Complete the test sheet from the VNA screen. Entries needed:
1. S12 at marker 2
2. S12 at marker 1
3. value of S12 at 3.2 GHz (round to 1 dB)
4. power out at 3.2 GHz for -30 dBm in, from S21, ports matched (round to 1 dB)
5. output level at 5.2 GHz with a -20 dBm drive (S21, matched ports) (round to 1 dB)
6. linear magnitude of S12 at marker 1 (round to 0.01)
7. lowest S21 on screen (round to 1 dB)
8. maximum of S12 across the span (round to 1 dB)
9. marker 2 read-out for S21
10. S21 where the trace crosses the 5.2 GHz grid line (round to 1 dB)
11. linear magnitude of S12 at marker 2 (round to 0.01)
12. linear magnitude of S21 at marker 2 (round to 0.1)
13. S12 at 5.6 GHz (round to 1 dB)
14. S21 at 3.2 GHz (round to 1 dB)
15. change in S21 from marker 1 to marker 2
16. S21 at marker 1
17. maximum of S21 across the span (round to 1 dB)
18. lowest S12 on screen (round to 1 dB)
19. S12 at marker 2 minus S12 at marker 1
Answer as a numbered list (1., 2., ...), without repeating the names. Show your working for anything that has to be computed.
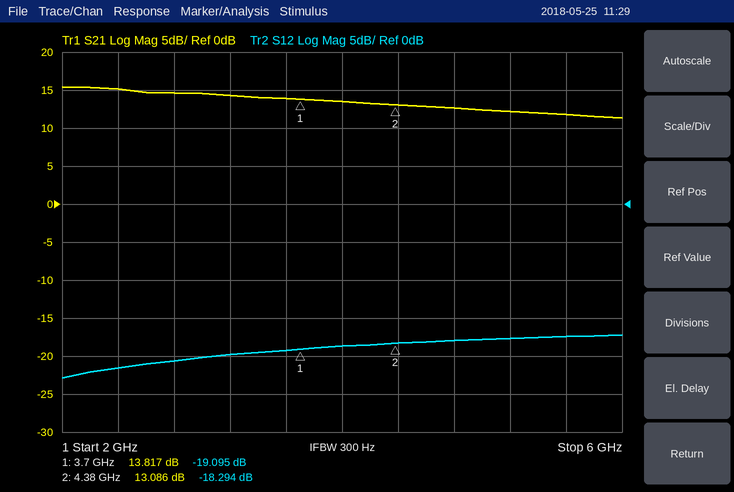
1. -18.294 dB
2. -19.095 dB
3. -20 dB
4. -30 dBm + (14 dB) = -16 dBm
5. -20 dBm + (12 dB) = -8 dBm
6. 10^(-19.095/20) ≈ 0.11
7. 11 dB
8. -17 dB
9. 13.086 dB
10. 12 dB
11. 10^(-18.294/20) ≈ 0.12
12. 10^(13.086/20) ≈ 4.5
13. -17 dB
14. 14 dB
15. 13.086 − (13.817) = -0.731 dB
16. 13.817 dB
17. 15 dB
18. -23 dB
19. -18.294 − (-19.095) = 0.801 dB
